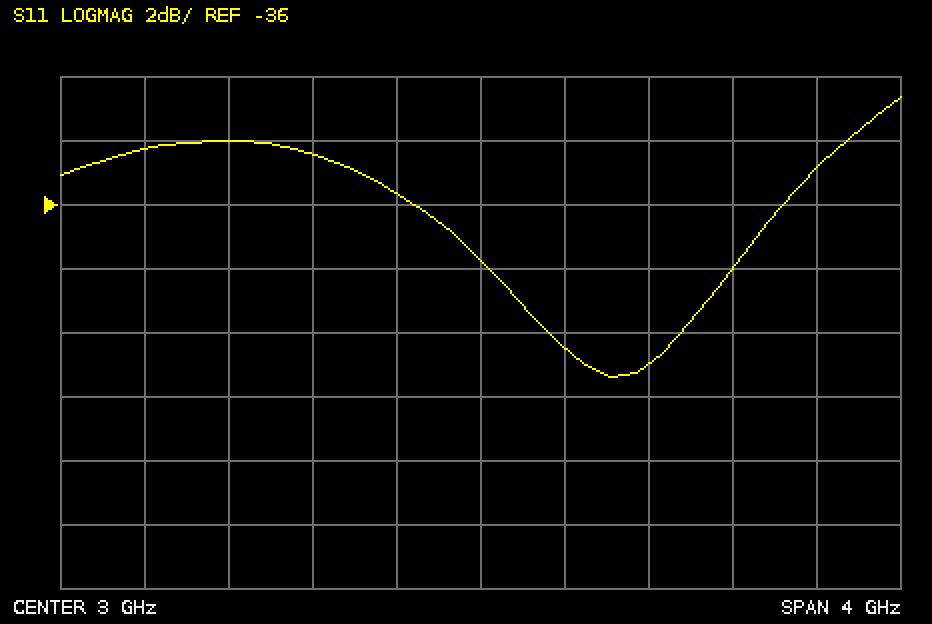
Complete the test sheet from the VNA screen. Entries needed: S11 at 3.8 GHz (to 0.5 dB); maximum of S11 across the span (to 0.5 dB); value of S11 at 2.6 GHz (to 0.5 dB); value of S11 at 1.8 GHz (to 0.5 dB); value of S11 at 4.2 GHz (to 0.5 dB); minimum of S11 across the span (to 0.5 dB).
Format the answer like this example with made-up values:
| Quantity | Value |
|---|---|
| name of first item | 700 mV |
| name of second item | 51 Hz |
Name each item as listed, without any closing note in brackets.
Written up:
| Quantity | Value |
|---|---|
| S11 at 3.8 GHz | -41.0 dB |
| maximum of S11 across the span | -32.5 dB |
| value of S11 at 2.6 GHz | -35.5 dB |
| value of S11 at 1.8 GHz | -34.0 dB |
| value of S11 at 4.2 GHz | -38.0 dB |
| minimum of S11 across the span | -41.5 dB |
